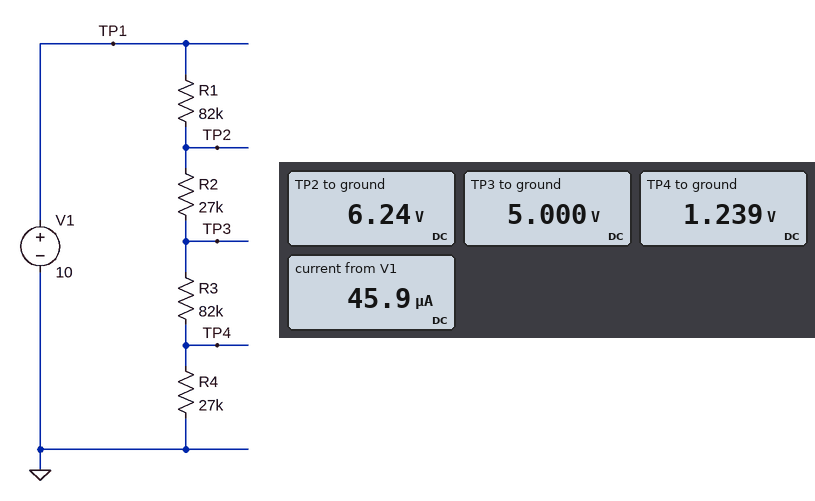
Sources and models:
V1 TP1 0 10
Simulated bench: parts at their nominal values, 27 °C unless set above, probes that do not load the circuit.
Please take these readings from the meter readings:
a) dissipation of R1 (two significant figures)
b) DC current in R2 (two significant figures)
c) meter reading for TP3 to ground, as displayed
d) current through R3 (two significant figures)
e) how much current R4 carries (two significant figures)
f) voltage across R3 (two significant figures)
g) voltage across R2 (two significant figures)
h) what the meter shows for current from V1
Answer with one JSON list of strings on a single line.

["170 µW", "46 µA", "5.000 V", "46 µA", "46 µA", "3.8 V", "1.2 V", "45.9 µA"]
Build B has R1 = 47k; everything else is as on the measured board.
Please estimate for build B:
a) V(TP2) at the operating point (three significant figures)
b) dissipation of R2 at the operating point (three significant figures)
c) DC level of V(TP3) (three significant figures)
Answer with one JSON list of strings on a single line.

["7.43 V", "80.6 µW", "5.96 V"]
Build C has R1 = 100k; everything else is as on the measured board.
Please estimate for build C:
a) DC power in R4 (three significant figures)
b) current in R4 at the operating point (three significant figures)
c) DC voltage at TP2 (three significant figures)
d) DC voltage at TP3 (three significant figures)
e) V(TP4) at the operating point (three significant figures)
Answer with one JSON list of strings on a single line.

["48.5 µW", "42.4 µA", "5.76 V", "4.62 V", "1.14 V"]
